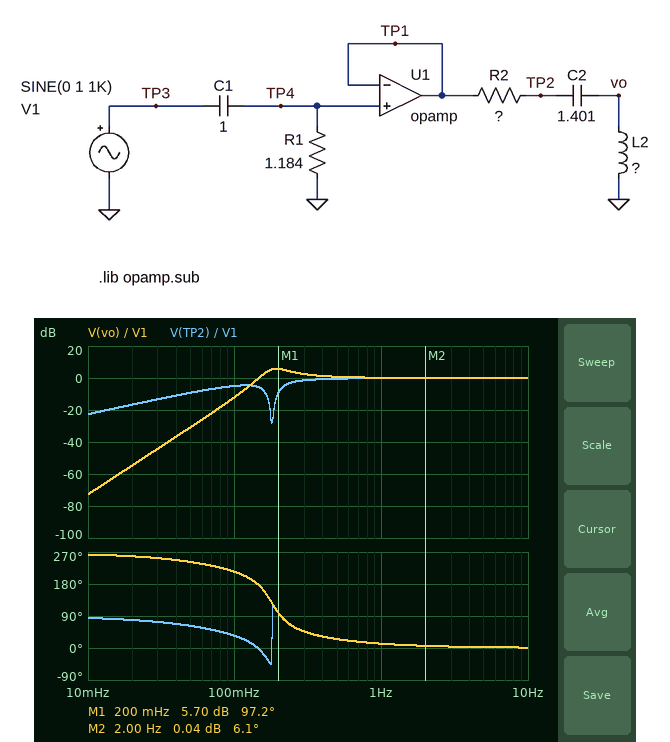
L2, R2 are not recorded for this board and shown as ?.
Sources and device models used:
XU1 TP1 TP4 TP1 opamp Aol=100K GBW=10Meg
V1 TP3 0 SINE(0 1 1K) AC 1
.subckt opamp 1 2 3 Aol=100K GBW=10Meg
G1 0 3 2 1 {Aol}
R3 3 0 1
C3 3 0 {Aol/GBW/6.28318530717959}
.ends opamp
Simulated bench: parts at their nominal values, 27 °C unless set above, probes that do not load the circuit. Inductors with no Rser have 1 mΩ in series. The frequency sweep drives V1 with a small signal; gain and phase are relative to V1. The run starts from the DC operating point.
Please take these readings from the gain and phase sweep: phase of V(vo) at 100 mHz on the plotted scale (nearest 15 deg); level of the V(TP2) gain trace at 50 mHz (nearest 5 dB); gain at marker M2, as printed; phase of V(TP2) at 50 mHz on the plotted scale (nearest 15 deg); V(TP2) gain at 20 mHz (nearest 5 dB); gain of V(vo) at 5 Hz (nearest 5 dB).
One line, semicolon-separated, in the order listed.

210 deg; -10 dB; 0.04 dB; 60 deg; -15 dB; 0 dB
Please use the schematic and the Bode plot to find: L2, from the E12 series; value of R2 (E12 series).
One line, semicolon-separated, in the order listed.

560 mH; 0.27 Ω
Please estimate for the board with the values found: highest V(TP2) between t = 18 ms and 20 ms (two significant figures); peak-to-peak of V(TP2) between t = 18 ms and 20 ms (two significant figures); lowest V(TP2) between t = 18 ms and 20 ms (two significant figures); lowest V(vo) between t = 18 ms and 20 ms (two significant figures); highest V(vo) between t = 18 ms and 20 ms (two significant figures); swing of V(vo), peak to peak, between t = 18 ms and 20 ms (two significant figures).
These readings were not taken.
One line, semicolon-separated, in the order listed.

1.0 V; 2.0 V; -1.0 V; -1.0 V; 1.0 V; 2.0 V
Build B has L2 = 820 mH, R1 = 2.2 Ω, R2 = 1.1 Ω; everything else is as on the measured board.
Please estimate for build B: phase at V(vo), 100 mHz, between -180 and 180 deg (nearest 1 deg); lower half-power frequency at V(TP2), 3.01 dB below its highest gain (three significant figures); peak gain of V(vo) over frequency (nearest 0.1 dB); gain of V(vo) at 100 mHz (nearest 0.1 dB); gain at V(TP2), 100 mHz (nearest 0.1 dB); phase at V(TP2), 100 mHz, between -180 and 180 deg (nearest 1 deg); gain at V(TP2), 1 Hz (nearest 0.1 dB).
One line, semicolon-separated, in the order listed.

155 deg; 300 mHz; 0 dB; -9.6 dB; -8.0 dB; -25 deg; -0.2 dB
